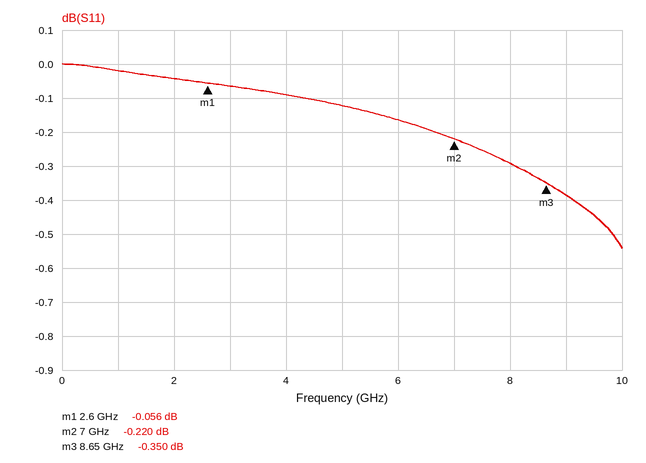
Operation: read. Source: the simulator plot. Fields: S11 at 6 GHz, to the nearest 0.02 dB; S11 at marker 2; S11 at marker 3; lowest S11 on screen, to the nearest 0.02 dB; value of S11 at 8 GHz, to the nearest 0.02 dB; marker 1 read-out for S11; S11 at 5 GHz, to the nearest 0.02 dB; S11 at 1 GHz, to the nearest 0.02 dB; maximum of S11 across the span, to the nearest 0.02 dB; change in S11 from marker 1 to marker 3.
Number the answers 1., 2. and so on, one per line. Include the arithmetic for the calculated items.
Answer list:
1. -0.16 dB
2. -0.220 dB
3. -0.350 dB
4. -0.54 dB
5. -0.30 dB
6. -0.056 dB
7. -0.12 dB
8. -0.02 dB
9. 0.00 dB
10. -0.35 − (-0.056) = -0.294 dB
